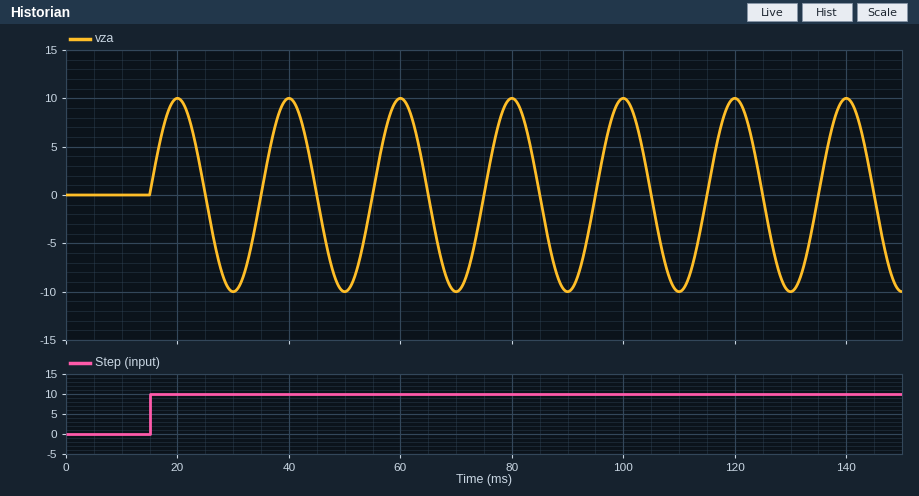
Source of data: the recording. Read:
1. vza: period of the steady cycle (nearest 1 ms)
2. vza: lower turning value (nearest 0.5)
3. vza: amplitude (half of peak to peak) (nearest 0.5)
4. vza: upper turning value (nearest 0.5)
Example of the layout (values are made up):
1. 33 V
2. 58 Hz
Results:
1. 20 ms
2. -10.0
3. 10.0
4. 10.0
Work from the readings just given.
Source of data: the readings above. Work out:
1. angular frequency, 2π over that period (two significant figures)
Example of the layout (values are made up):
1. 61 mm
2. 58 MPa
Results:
1. 0.31 rad/ms
